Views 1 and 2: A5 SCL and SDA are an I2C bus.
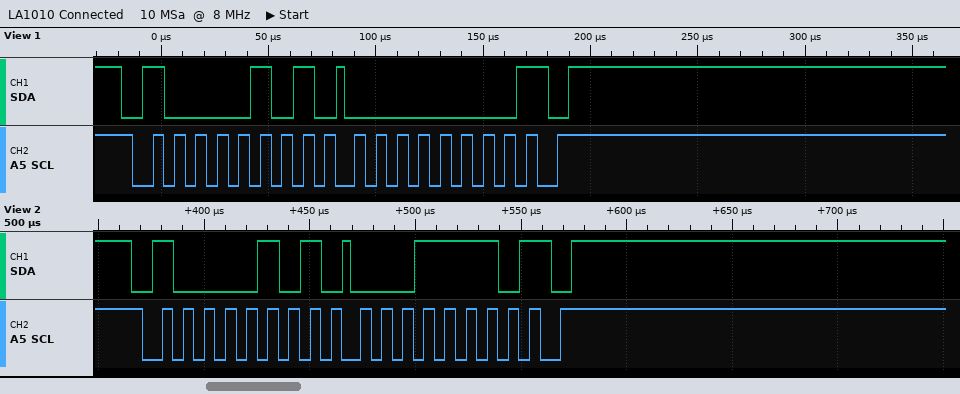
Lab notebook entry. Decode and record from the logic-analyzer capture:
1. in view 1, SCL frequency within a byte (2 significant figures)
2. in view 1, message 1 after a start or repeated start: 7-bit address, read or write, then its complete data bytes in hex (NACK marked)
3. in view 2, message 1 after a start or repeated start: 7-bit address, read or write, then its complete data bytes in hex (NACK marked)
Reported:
100 kHz
0x42 read: 00 NACK
0x42 read: 1E NACK
